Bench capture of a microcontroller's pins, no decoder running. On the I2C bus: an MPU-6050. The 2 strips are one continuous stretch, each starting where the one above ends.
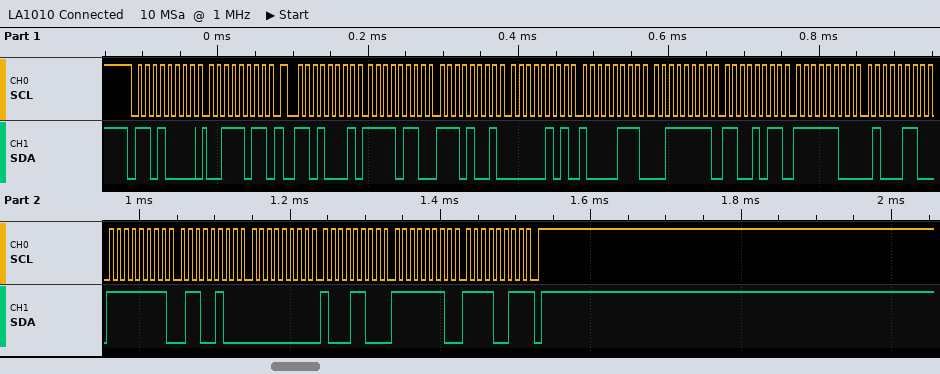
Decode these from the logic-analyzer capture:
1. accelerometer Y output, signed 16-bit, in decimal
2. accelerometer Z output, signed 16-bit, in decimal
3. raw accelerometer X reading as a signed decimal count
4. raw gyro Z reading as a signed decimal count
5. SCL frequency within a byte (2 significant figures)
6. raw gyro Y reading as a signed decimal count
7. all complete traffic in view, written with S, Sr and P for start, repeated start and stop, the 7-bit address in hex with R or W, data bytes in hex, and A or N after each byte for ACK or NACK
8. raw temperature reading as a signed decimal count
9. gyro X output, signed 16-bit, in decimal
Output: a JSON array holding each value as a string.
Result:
["1415", "16331", "-2327", "-269", "100 kHz", "140", "S 68W A 3B A Sr 68R A F6 A E9 A 05 A 87 A 3F A CB A FC A 46 A FF A 64 A 00 A 8C A FE A F3 N P", "-954", "-156"]
